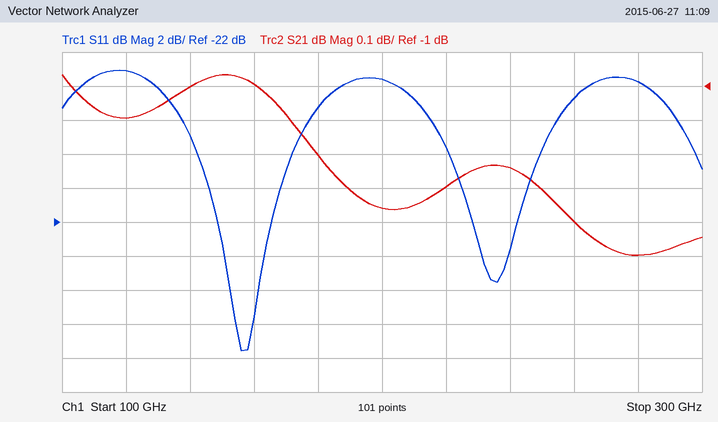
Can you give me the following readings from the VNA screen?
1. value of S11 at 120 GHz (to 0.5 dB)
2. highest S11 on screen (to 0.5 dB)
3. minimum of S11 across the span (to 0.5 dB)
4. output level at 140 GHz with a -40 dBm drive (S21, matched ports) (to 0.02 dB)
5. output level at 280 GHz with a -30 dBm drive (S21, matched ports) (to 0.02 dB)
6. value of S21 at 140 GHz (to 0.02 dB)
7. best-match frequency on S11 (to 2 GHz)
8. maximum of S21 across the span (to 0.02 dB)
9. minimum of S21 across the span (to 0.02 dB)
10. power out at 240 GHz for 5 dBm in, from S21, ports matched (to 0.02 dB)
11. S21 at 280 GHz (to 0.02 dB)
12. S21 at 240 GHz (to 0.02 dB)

-13.0 dB
-13.0 dB
-29.5 dB
-41.00 dBm
-31.50 dBm
-1.00 dB
156 GHz
-0.96 dB
-1.50 dB
3.76 dBm
-1.50 dB
-1.24 dB
